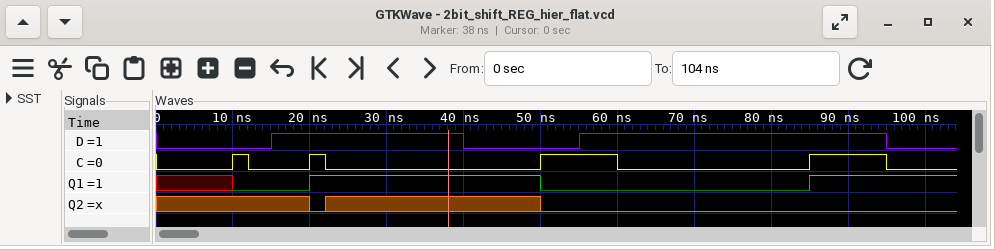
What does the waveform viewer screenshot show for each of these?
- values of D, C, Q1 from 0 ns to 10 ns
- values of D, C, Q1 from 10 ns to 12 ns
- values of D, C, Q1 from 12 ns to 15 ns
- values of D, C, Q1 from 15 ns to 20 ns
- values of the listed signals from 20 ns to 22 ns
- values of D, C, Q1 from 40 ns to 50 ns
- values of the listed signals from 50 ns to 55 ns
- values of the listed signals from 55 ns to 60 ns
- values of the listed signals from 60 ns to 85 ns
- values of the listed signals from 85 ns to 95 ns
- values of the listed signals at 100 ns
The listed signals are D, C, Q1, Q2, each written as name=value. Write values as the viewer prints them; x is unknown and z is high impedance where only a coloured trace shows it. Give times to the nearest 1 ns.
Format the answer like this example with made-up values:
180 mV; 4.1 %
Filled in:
D=0, C=0, Q1=x; D=0, C=1, Q1=0; D=0, C=0, Q1=0; D=1, C=0, Q1=0; D=1, C=1, Q1=1, Q2=0; D=0, C=0, Q1=1; D=0, C=1, Q1=0, Q2=0; D=1, C=1, Q1=0, Q2=0; D=1, C=0, Q1=0, Q2=0; D=1, C=1, Q1=1, Q2=0; D=0, C=0, Q1=1, Q2=0
